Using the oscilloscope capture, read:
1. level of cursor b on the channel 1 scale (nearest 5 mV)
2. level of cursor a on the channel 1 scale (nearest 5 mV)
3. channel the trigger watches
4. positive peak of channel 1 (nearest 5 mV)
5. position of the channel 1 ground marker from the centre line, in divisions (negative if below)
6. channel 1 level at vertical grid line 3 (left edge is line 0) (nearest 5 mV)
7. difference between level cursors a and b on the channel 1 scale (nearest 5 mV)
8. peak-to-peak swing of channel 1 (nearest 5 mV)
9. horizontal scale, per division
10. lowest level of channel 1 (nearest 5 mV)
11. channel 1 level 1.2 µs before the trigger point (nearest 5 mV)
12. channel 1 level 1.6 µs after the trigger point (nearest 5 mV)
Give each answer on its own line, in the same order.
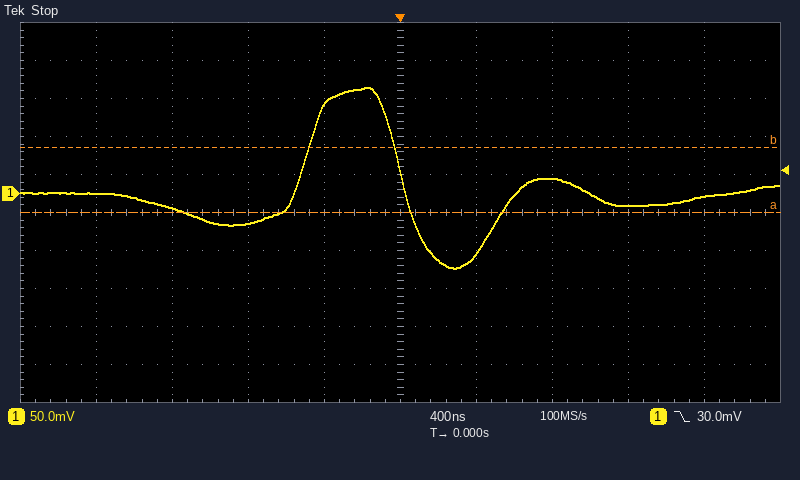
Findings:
60 mV
-25 mV
channel 1
140 mV
+0.5 div
-40 mV
85 mV
240 mV
400 ns
-100 mV
-20 mV
-5 mV
